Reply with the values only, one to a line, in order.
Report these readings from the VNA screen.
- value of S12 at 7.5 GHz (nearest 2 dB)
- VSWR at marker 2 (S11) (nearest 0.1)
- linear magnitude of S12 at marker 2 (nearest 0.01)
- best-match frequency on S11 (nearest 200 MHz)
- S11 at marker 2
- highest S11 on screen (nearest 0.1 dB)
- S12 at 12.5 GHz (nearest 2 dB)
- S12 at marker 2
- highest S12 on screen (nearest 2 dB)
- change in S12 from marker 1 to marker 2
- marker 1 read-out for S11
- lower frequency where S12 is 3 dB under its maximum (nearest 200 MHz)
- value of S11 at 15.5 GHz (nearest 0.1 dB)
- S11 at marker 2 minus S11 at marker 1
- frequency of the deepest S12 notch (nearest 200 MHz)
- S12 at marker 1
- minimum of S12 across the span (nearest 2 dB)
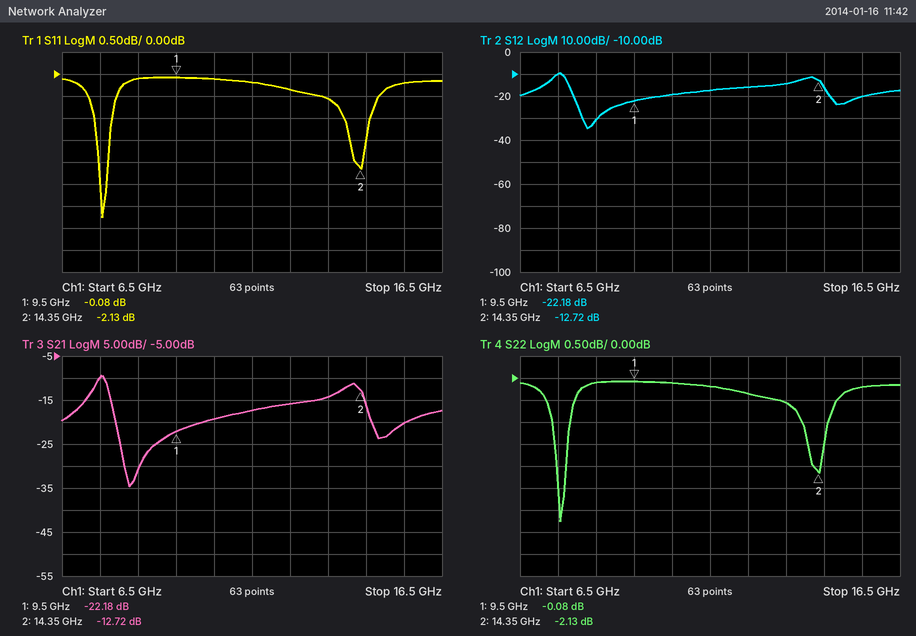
-10 dB
8.2
0.23
7.6 GHz
-2.13 dB
-0.1 dB
-16 dB
-12.72 dB
-10 dB
9.46 dB
-0.08 dB
7.4 GHz
-0.2 dB
-2.05 dB
8.2 GHz
-22.18 dB
-34 dB
